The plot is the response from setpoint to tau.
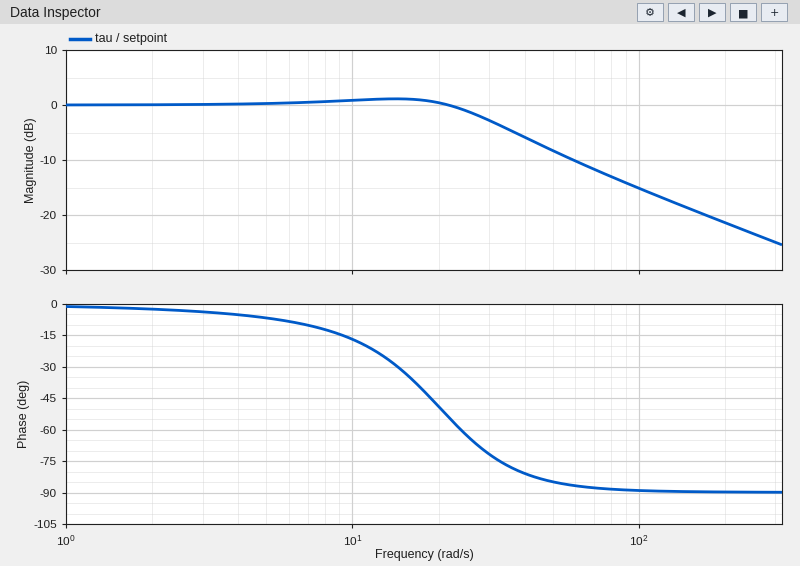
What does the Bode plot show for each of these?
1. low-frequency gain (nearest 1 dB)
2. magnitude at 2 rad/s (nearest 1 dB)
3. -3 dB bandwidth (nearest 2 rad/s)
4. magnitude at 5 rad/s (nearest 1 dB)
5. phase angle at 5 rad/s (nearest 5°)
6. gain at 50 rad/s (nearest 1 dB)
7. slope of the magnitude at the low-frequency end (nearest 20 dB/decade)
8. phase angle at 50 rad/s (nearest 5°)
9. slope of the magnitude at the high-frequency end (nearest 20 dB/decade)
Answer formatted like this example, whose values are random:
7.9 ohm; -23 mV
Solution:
0 dB; 0 dB; 30 rad/s; 0 dB; -5°; -8 dB; 0 dB/decade; -85°; -20 dB/decade
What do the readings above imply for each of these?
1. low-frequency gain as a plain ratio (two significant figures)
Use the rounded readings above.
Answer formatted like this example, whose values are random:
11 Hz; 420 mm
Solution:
1.0
